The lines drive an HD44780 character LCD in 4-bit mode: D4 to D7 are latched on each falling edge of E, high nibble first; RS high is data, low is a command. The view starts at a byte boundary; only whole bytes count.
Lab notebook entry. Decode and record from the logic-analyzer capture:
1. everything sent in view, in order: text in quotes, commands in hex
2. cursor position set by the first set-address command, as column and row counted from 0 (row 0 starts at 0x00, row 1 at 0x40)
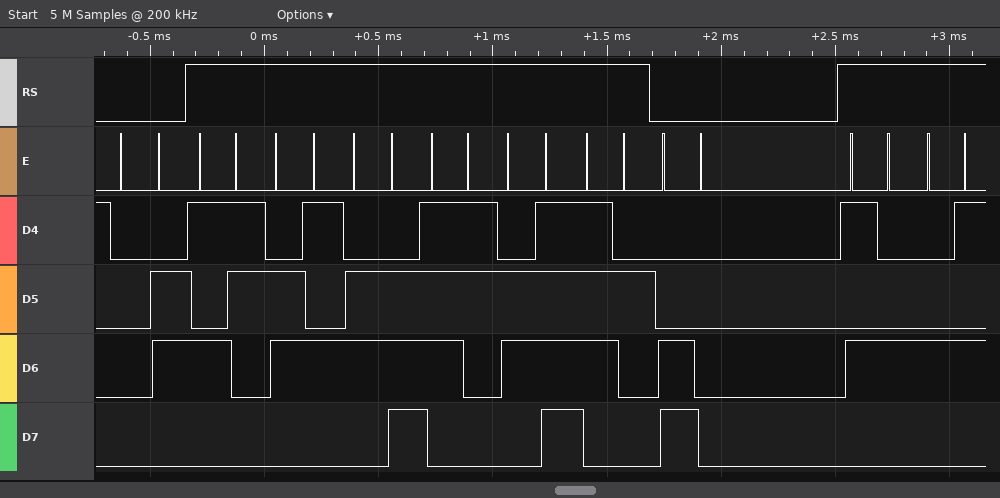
0x06 "Sensor" 0xC0 "TE"
column 0, row 1
